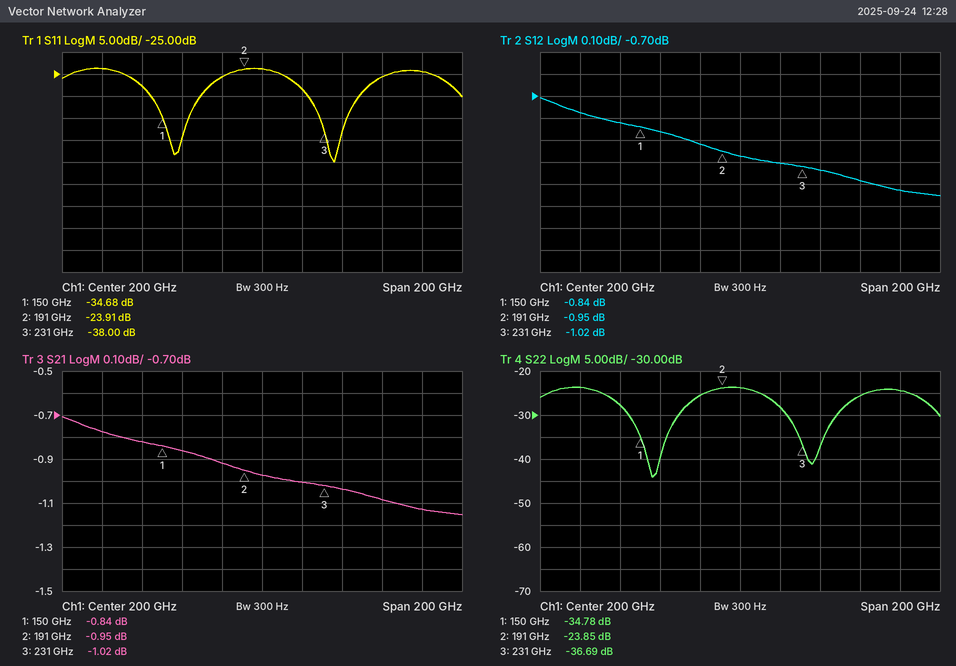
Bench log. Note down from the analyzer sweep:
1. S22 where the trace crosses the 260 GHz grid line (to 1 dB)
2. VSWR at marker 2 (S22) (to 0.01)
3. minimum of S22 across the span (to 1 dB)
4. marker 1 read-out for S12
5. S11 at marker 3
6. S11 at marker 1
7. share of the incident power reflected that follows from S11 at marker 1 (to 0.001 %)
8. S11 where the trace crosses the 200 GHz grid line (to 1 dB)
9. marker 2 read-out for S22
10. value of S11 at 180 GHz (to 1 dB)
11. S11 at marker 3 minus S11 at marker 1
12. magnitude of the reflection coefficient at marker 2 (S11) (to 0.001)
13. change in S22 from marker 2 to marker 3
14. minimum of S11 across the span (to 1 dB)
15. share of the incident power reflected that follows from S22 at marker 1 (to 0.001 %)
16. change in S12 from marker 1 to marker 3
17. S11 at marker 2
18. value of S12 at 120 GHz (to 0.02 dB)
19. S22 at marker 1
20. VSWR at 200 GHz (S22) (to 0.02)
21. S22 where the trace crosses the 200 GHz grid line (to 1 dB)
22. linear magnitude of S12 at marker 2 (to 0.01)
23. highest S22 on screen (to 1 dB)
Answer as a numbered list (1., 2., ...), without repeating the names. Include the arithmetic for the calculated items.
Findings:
1. -26 dB
2. (1 + 0.0642)/(1 − 0.0642) ≈ 1.14
3. -44 dB
4. -0.84 dB
5. -38.00 dB
6. -34.68 dB
7. 10^(-34.68/10) ≈ 0.034 %
8. -24 dB
9. -23.85 dB
10. -26 dB
11. -38 − (-34.68) = -3.32 dB
12. 10^(-23.91/20) ≈ 0.064
13. -36.69 − (-23.85) = -12.84 dB
14. -45 dB
15. 10^(-34.78/10) ≈ 0.033 %
16. -1.02 − (-0.84) = -0.18 dB
17. -23.91 dB
18. -0.78 dB
19. -34.78 dB
20. |Γ| = 10^(-24/20) = 0.0631; VSWR = (1 + 0.0631)/(1 − 0.0631) ≈ 1.13, so 1.14 to the nearest 0.02
21. -24 dB
22. 10^(-0.95/20) ≈ 0.90
23. -24 dB
